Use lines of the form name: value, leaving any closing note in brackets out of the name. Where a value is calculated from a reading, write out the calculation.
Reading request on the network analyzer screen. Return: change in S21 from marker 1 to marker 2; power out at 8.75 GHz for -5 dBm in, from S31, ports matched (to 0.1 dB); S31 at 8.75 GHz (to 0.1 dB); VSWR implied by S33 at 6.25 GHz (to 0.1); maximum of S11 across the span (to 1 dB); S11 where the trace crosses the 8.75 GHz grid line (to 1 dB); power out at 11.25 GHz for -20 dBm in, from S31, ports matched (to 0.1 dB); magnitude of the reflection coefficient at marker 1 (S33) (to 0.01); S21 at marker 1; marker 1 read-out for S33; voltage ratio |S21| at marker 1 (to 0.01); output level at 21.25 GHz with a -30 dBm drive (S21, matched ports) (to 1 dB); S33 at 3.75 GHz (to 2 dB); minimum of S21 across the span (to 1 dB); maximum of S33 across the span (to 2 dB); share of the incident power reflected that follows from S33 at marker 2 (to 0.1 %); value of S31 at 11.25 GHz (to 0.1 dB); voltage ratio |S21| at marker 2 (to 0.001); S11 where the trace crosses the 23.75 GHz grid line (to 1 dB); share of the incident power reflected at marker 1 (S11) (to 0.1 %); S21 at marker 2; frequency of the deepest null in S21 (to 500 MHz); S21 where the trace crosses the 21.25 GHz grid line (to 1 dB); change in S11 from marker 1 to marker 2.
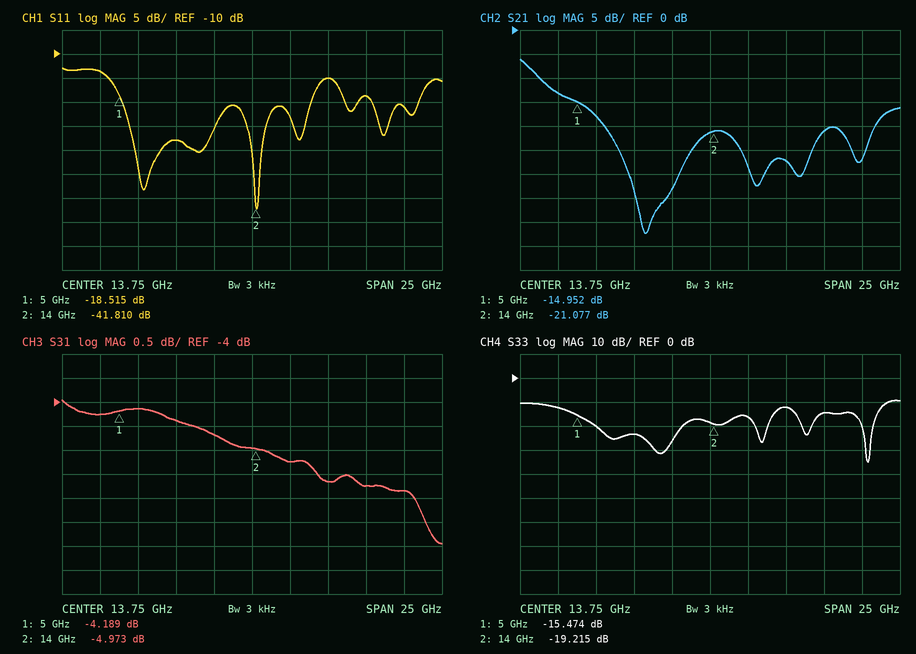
change in S21 from marker 1 to marker 2: -21.077 − (-14.952) = -6.125 dB
power out at 8.75 GHz for -5 dBm in, from S31, ports matched: -5 dBm + (-4.4 dB) = -9.4 dBm
S31 at 8.75 GHz: -4.4 dB
VSWR implied by S33 at 6.25 GHz: |Γ| = 10^(-20/20) = 0.1000; VSWR = (1 + 0.1000)/(1 − 0.1000) ≈ 1.2
maximum of S11 across the span: -13 dB
S11 where the trace crosses the 8.75 GHz grid line: -28 dB
power out at 11.25 GHz for -20 dBm in, from S31, ports matched: -20 dBm + (-4.7 dB) = -24.7 dBm
magnitude of the reflection coefficient at marker 1 (S33): 10^(-15.474/20) ≈ 0.17
S21 at marker 1: -14.952 dB
marker 1 read-out for S33: -15.474 dB
voltage ratio |S21| at marker 1: 10^(-14.952/20) ≈ 0.18
output level at 21.25 GHz with a -30 dBm drive (S21, matched ports): -30 dBm + (-21 dB) = -51 dBm
S33 at 3.75 GHz: -12 dB
minimum of S21 across the span: -42 dB
maximum of S33 across the span: -10 dB
share of the incident power reflected that follows from S33 at marker 2: 10^(-19.215/10) ≈ 1.2 %
value of S31 at 11.25 GHz: -4.7 dB
voltage ratio |S21| at marker 2: 10^(-21.077/20) ≈ 0.088
S11 where the trace crosses the 23.75 GHz grid line: -21 dB
share of the incident power reflected at marker 1 (S11): 10^(-18.515/10) ≈ 1.4 %
S21 at marker 2: -21.077 dB
frequency of the deepest null in S21: 9.5 GHz
S21 where the trace crosses the 21.25 GHz grid line: -21 dB
change in S11 from marker 1 to marker 2: -41.81 − (-18.515) = -23.295 dB
